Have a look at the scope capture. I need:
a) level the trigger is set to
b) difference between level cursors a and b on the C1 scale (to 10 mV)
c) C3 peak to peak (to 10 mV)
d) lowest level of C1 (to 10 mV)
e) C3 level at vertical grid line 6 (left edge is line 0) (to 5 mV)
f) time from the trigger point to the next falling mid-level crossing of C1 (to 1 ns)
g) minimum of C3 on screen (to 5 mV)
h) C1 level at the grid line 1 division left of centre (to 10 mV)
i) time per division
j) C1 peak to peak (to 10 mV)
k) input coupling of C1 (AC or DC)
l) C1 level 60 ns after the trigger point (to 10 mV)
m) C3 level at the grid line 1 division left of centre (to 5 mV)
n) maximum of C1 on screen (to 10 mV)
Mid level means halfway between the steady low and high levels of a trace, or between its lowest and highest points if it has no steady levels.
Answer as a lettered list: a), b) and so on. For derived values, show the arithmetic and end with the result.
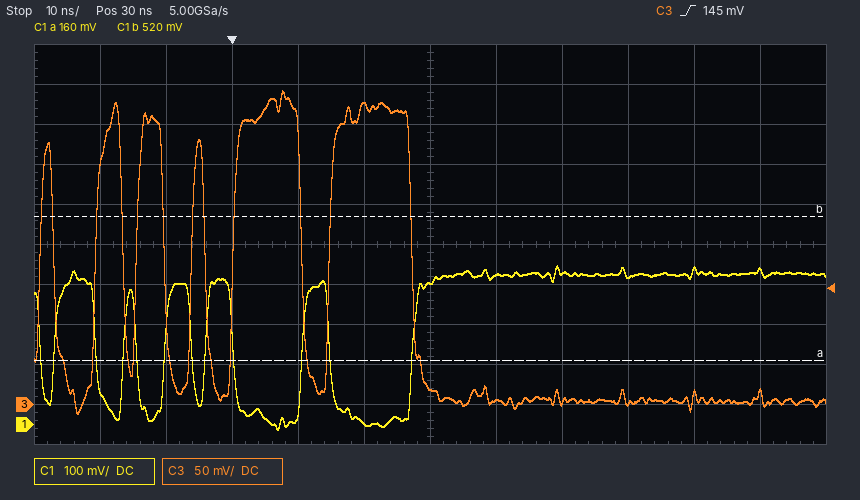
a) 145 mV
b) 360 mV
c) 400 mV
d) -10 mV
e) 20 mV
f) 15 ns
g) -10 mV
h) 0 mV
i) 10 ns
j) 400 mV − (-10 mV) = 410 mV
k) DC
l) 370 mV
m) 375 mV
n) 400 mV
